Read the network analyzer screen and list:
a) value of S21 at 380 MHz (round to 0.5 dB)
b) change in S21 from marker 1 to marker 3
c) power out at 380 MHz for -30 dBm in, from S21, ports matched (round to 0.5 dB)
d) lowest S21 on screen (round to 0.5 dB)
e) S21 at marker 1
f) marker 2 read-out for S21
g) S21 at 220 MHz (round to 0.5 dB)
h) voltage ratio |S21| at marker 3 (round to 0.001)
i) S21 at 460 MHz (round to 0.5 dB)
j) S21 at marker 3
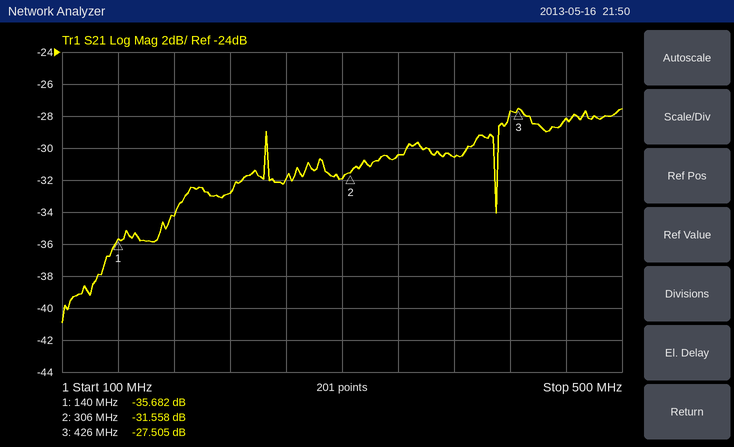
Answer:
-30.5 dB
8.177 dB
-60.5 dBm
-41.0 dB
-35.682 dB
-31.558 dB
-33.0 dB
0.042
-28.0 dB
-27.505 dB
